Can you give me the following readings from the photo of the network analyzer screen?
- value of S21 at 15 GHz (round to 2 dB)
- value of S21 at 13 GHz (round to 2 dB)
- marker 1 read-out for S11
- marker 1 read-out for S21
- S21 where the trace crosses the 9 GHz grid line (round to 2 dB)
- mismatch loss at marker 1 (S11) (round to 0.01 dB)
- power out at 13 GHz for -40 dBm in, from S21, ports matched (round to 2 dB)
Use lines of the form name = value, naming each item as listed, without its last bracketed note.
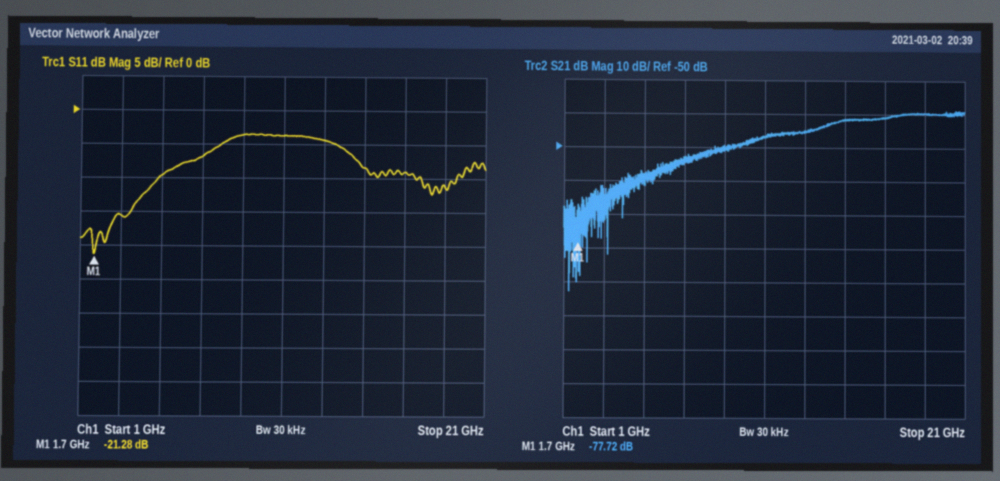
value of S21 at 15 GHz = -42 dB
value of S21 at 13 GHz = -46 dB
marker 1 read-out for S11 = -21.28 dB
marker 1 read-out for S21 = -77.72 dB
S21 where the trace crosses the 9 GHz grid line = -50 dB
mismatch loss at marker 1 (S11) = 0.03 dB
power out at 13 GHz for -40 dBm in, from S21, ports matched = -86 dBm
